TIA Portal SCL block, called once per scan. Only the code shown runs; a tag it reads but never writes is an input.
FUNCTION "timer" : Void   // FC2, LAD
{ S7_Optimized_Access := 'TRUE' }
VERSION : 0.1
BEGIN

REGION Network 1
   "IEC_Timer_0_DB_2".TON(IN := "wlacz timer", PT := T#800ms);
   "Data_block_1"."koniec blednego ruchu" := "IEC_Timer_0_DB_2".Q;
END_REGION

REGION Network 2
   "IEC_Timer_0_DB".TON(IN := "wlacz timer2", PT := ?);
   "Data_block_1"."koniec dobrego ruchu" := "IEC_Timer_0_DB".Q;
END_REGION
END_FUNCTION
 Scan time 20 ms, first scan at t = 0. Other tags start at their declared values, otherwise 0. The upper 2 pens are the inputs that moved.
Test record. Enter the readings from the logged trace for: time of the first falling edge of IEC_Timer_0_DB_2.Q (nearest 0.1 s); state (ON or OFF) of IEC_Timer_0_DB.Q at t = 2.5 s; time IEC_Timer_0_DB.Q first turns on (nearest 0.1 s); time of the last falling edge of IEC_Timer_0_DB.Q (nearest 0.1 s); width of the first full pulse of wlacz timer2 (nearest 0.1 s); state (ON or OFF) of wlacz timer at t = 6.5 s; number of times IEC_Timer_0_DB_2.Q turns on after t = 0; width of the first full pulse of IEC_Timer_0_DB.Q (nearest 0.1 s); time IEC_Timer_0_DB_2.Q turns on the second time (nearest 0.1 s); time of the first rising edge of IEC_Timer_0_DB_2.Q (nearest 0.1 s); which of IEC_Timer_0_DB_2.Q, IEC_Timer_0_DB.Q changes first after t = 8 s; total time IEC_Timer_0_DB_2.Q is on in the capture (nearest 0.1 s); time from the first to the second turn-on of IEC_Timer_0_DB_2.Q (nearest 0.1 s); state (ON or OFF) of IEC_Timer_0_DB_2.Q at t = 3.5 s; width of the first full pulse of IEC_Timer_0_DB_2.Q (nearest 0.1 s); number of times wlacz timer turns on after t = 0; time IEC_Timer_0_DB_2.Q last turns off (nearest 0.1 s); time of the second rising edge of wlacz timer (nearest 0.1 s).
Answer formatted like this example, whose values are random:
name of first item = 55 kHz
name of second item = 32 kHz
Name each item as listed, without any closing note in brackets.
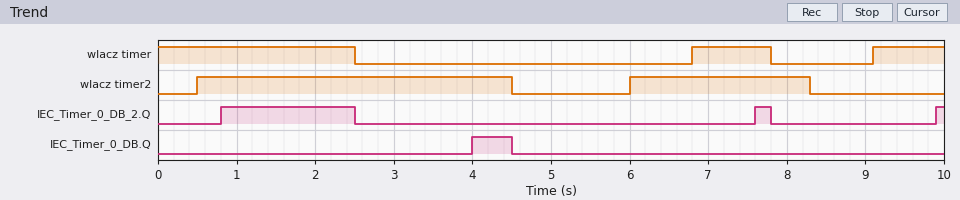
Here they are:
time of the first falling edge of IEC_Timer_0_DB_2.Q = 2.5 s
state (ON or OFF) of IEC_Timer_0_DB.Q at t = 2.5 s = OFF
time IEC_Timer_0_DB.Q first turns on = 4.0 s
time of the last falling edge of IEC_Timer_0_DB.Q = 4.5 s
width of the first full pulse of wlacz timer2 = 4.0 s
state (ON or OFF) of wlacz timer at t = 6.5 s = OFF
number of times IEC_Timer_0_DB_2.Q turns on after t = 0 = 3
width of the first full pulse of IEC_Timer_0_DB.Q = 0.5 s
time IEC_Timer_0_DB_2.Q turns on the second time = 7.6 s
time of the first rising edge of IEC_Timer_0_DB_2.Q = 0.8 s
which of IEC_Timer_0_DB_2.Q, IEC_Timer_0_DB.Q changes first after t = 8 s = IEC_Timer_0_DB_2.Q
total time IEC_Timer_0_DB_2.Q is on in the capture = 2.0 s
time from the first to the second turn-on of IEC_Timer_0_DB_2.Q = 6.8 s
state (ON or OFF) of IEC_Timer_0_DB_2.Q at t = 3.5 s = OFF
width of the first full pulse of IEC_Timer_0_DB_2.Q = 1.7 s
number of times wlacz timer turns on after t = 0 = 2
time IEC_Timer_0_DB_2.Q last turns off = 7.8 s
time of the second rising edge of wlacz timer = 9.1 s
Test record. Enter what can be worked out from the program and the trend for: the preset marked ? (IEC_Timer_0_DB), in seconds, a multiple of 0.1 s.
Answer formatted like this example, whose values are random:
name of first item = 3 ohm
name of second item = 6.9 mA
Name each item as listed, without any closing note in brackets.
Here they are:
the preset marked ? (IEC_Timer_0_DB), in seconds, a multiple of 0.1 s = 3.5 s
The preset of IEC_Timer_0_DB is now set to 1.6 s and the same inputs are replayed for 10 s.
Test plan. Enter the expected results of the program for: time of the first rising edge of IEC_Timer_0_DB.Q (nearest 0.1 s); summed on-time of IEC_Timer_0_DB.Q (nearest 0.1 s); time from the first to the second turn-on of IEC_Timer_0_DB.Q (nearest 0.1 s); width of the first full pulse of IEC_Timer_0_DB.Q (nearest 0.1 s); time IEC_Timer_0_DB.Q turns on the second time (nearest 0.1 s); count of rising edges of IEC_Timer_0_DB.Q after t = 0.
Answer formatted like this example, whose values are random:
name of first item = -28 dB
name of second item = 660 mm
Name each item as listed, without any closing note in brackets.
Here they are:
time of the first rising edge of IEC_Timer_0_DB.Q = 2.1 s
summed on-time of IEC_Timer_0_DB.Q = 3.1 s
time from the first to the second turn-on of IEC_Timer_0_DB.Q = 5.5 s
width of the first full pulse of IEC_Timer_0_DB.Q = 2.4 s
time IEC_Timer_0_DB.Q turns on the second time = 7.6 s
count of rising edges of IEC_Timer_0_DB.Q after t = 0 = 2
